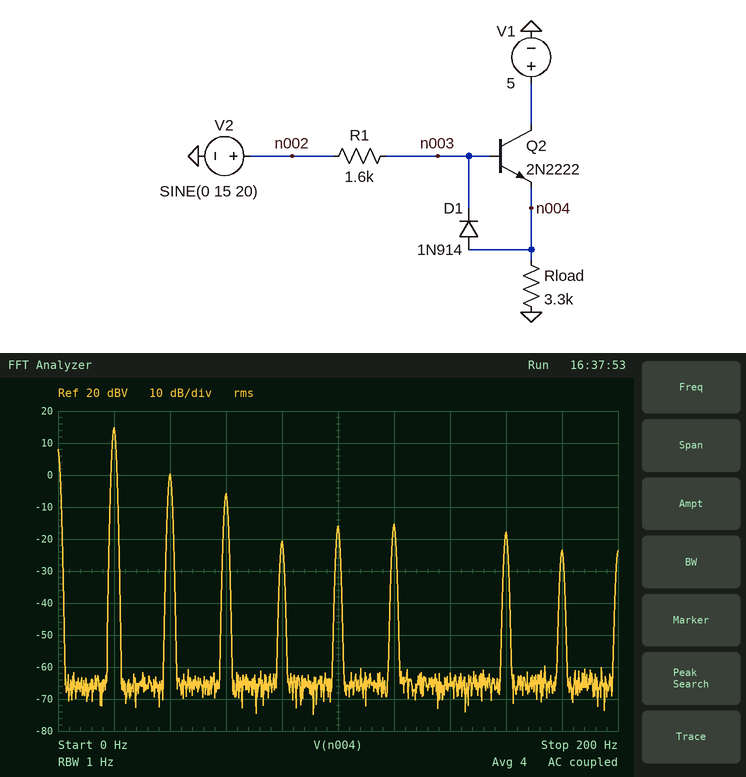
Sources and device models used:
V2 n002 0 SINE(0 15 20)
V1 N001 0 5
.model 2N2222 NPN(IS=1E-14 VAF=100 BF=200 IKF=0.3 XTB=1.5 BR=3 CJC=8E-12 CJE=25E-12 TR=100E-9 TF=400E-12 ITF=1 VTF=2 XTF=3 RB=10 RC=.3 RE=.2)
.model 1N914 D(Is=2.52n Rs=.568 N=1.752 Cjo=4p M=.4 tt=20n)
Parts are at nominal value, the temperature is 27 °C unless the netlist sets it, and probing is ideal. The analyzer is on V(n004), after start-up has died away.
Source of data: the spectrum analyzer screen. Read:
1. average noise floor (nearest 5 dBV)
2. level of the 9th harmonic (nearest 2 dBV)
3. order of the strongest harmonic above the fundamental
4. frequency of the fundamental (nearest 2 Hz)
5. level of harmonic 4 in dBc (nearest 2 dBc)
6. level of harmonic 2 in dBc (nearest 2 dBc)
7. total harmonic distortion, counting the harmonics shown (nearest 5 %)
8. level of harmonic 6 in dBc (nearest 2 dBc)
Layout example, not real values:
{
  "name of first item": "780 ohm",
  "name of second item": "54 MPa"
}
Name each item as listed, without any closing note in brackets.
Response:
{
  "average noise floor": "-65 dBV",
  "level of the 9th harmonic": "-24 dBV",
  "order of the strongest harmonic above the fundamental": "2",
  "frequency of the fundamental": "20 Hz",
  "level of harmonic 4 in dBc": "-36 dBc",
  "level of harmonic 2 in dBc": "-14 dBc",
  "total harmonic distortion, counting the harmonics shown": "20 %",
  "level of harmonic 6 in dBc": "-30 dBc"
}
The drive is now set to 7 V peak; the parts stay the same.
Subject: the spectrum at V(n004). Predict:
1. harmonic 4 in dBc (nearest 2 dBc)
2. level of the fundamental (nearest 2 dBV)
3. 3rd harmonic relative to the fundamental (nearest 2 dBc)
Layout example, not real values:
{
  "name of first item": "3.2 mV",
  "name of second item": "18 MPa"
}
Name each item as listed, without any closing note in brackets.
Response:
{
  "harmonic 4 in dBc": "-26 dBc",
  "level of the fundamental": "10 dBV",
  "3rd harmonic relative to the fundamental": "-42 dBc"
}
